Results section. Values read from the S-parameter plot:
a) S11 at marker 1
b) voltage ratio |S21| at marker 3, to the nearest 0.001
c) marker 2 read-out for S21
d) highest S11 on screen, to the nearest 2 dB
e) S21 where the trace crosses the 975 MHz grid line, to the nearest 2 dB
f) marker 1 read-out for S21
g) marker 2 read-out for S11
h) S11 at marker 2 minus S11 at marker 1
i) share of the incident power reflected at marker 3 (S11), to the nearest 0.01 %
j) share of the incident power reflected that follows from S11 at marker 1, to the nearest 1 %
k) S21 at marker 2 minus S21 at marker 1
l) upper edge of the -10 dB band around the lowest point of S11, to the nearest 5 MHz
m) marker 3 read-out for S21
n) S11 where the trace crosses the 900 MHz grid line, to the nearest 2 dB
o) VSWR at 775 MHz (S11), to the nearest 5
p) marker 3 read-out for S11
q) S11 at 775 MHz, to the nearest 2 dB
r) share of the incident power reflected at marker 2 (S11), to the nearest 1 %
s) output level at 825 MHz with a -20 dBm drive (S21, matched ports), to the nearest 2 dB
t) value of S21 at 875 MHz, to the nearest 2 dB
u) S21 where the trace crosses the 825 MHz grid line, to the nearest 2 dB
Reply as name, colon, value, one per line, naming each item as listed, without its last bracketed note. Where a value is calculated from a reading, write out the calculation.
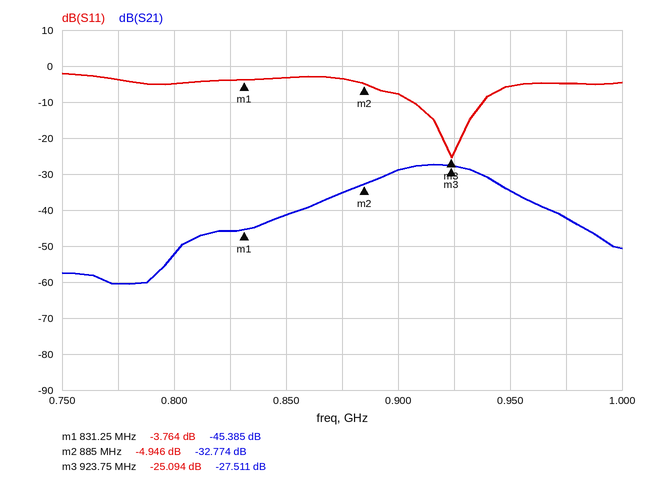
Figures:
S11 at marker 1: -3.764 dB
voltage ratio |S21| at marker 3, to the nearest 0.001: 10^(-27.511/20) ≈ 0.042
marker 2 read-out for S21: -32.774 dB
highest S11 on screen, to the nearest 2 dB: -2 dB
S21 where the trace crosses the 975 MHz grid line, to the nearest 2 dB: -42 dB
marker 1 read-out for S21: -45.385 dB
marker 2 read-out for S11: -4.946 dB
S11 at marker 2 minus S11 at marker 1: -4.946 − (-3.764) = -1.182 dB
share of the incident power reflected at marker 3 (S11), to the nearest 0.01 %: 10^(-25.094/10) ≈ 0.31 %
share of the incident power reflected that follows from S11 at marker 1, to the nearest 1 %: 10^(-3.764/10) ≈ 42 %
S21 at marker 2 minus S21 at marker 1: -32.774 − (-45.385) = 12.611 dB
upper edge of the -10 dB band around the lowest point of S11, to the nearest 5 MHz: 940 MHz
marker 3 read-out for S21: -27.511 dB
S11 where the trace crosses the 900 MHz grid line, to the nearest 2 dB: -8 dB
VSWR at 775 MHz (S11), to the nearest 5: |Γ| = 10^(-4/20) = 0.6310; VSWR = (1 + 0.6310)/(1 − 0.6310) ≈ 4.42, so 5 to the nearest 5
marker 3 read-out for S11: -25.094 dB
S11 at 775 MHz, to the nearest 2 dB: -4 dB
share of the incident power reflected at marker 2 (S11), to the nearest 1 %: 10^(-4.946/10) ≈ 32 %
output level at 825 MHz with a -20 dBm drive (S21, matched ports), to the nearest 2 dB: -20 dBm + (-46 dB) = -66 dBm
value of S21 at 875 MHz, to the nearest 2 dB: -36 dB
S21 where the trace crosses the 825 MHz grid line, to the nearest 2 dB: -46 dB
